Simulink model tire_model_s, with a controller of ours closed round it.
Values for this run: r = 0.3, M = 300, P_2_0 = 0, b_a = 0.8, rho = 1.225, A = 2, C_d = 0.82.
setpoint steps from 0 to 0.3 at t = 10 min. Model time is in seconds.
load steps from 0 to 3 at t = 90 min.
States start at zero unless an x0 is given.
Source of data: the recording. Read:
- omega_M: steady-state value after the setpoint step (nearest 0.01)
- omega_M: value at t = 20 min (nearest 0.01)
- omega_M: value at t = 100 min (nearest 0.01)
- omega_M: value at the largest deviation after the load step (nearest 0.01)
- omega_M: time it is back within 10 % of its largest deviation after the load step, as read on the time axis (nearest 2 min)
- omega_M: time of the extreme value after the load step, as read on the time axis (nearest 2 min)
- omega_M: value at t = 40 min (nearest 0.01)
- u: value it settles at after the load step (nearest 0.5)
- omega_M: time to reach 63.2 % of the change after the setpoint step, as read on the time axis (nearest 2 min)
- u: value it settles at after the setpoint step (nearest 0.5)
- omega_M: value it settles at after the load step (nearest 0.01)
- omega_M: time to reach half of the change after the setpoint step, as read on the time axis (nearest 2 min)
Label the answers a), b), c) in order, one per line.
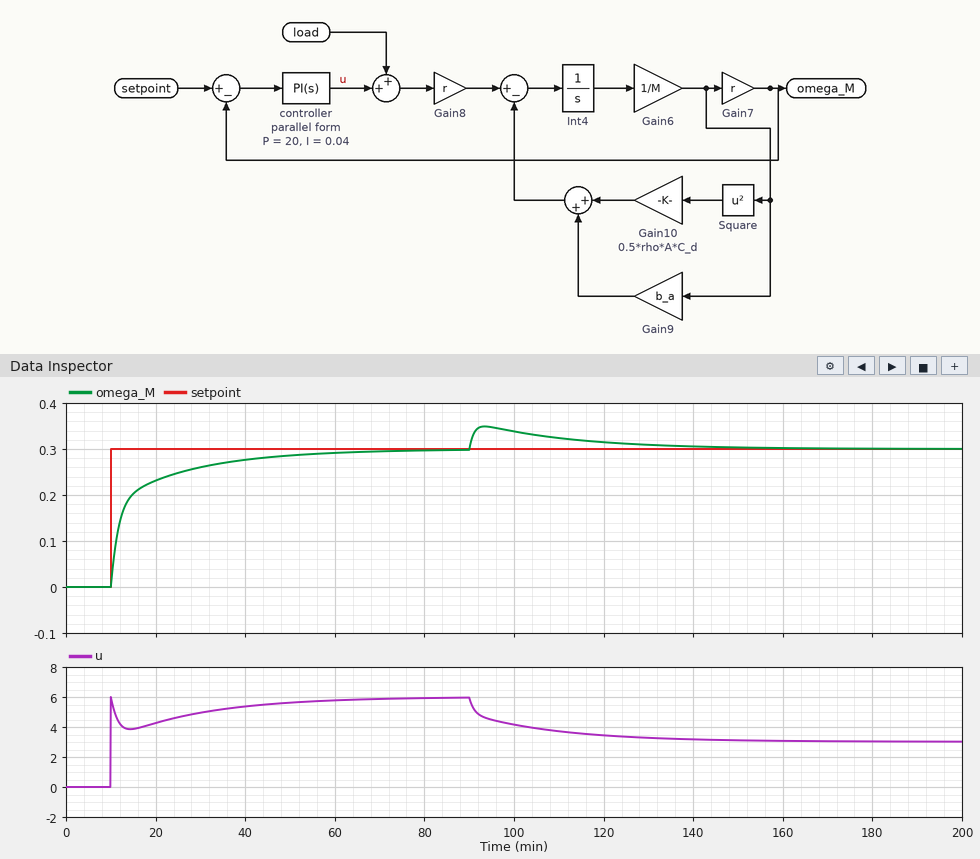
a) 0.30
b) 0.23
c) 0.34
d) 0.35
e) 142 min
f) 94 min
g) 0.28
h) 3.0
i) 14 min
j) 6.0
k) 0.30
l) 12 min
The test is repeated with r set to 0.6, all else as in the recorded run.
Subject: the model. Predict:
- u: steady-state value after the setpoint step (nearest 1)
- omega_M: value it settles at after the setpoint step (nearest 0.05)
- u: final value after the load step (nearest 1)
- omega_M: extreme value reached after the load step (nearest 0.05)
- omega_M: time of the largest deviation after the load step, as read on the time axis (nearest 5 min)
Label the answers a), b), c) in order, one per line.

a) 1
b) 0.30
c) -2
d) 0.40
e) 90 min
